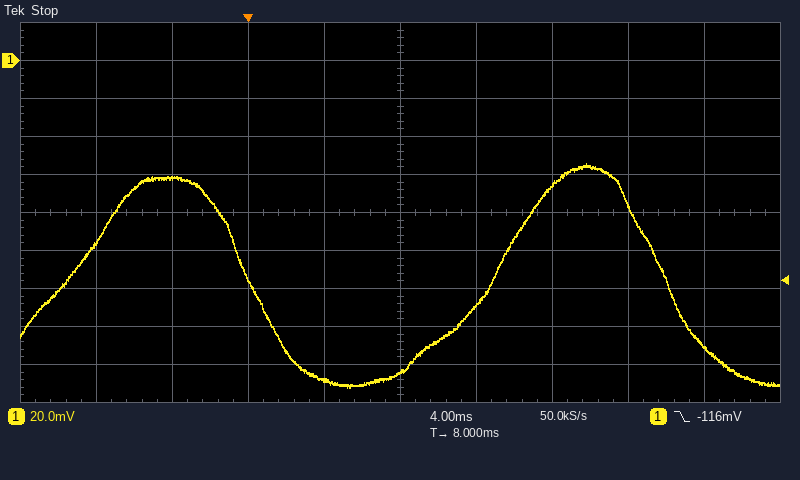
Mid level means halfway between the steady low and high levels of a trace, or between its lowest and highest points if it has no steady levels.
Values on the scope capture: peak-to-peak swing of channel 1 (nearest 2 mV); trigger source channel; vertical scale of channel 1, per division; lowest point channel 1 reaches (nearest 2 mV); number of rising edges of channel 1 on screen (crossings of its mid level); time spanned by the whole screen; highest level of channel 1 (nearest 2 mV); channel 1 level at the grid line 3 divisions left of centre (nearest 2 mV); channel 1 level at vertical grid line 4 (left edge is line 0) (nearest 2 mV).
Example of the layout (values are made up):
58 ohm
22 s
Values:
118 mV
channel 1
20 mV
-172 mV
2
40 ms
-54 mV
-62 mV
-168 mV
